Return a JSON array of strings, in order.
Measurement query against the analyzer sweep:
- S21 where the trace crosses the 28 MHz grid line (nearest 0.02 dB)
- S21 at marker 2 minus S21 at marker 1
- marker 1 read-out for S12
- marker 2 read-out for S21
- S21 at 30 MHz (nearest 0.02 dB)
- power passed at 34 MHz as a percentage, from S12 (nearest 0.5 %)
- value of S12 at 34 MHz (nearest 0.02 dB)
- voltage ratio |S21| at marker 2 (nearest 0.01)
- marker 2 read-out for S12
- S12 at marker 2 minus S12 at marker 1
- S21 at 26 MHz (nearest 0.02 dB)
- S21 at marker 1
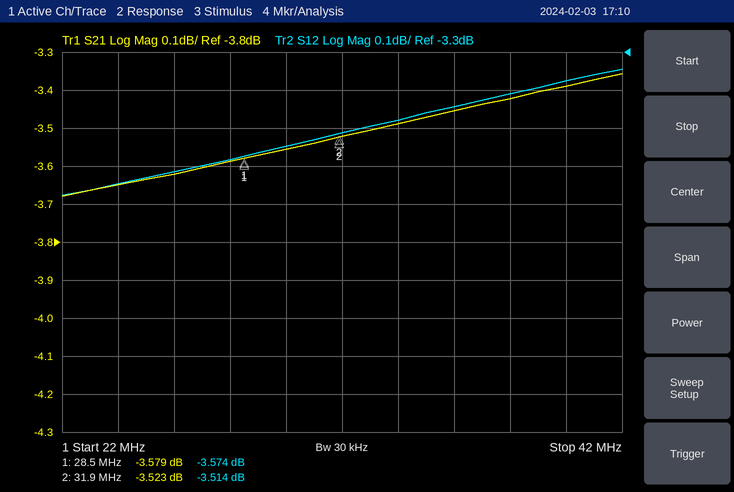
["-3.58 dB", "0.056 dB", "-3.574 dB", "-3.523 dB", "-3.56 dB", "45.0 %", "-3.48 dB", "0.67", "-3.514 dB", "0.060 dB", "-3.62 dB", "-3.579 dB"]
